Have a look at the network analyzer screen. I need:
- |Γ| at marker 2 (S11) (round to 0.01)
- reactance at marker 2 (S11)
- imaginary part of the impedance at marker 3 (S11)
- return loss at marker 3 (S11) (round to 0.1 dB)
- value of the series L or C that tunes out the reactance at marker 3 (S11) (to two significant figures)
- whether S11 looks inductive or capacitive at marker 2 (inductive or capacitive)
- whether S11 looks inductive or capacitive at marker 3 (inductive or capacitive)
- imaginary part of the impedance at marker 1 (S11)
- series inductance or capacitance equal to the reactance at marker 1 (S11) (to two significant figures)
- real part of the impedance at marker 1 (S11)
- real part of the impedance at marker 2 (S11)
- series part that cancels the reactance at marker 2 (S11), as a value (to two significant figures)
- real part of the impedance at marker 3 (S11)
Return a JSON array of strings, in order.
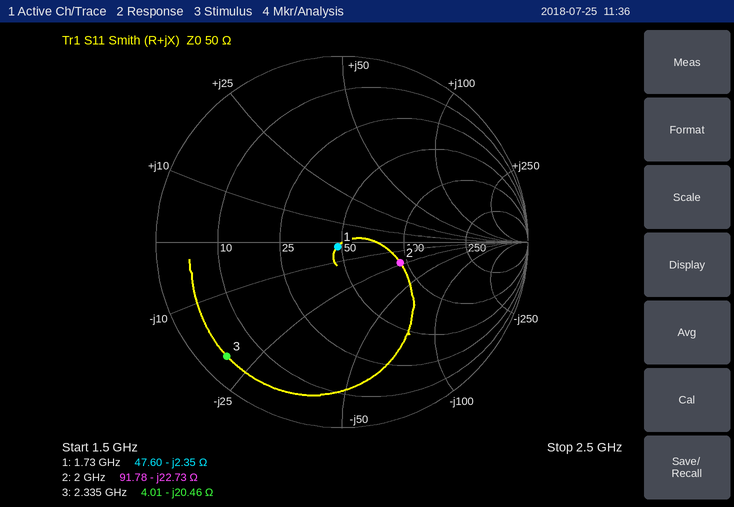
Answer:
["0.33", "-22.73 Ω", "-20.46 Ω", "1.2 dB", "1.4 nH", "capacitive", "capacitive", "-2.35 Ω", "39 pF", "47.60 Ω", "91.78 Ω", "1.8 nH", "4.01 Ω"]
